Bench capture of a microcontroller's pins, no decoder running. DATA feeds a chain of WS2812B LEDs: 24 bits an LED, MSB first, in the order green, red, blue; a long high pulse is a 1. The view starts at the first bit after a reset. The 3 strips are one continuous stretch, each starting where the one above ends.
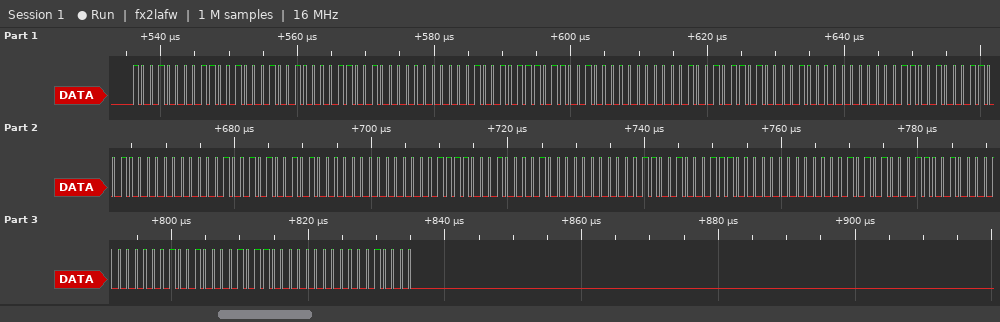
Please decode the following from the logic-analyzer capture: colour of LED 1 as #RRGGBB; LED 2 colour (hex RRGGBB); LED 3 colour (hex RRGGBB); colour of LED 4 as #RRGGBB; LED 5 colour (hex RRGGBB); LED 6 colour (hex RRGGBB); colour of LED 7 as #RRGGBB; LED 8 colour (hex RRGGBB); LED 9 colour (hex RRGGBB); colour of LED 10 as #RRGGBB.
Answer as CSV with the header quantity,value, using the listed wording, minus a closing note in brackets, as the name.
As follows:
quantity,value
colour of LED 1 as #RRGGBB,#C89090
LED 2 colour,#00C897
LED 3 colour,#00644B
colour of LED 4 as #RRGGBB,#004232
LED 5 colour,#003225
LED 6 colour,#00281E
colour of LED 7 as #RRGGBB,#002119
LED 8 colour,#001C15
LED 9 colour,#001912
colour of LED 10 as #RRGGBB,#001610
